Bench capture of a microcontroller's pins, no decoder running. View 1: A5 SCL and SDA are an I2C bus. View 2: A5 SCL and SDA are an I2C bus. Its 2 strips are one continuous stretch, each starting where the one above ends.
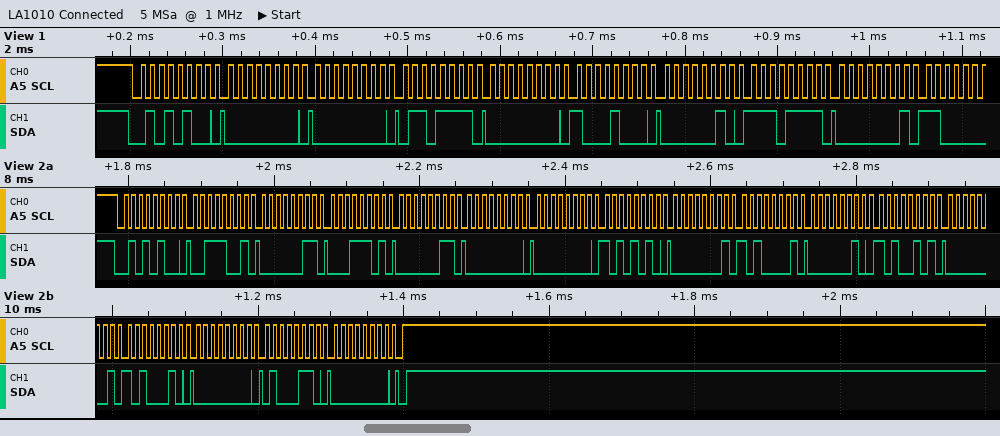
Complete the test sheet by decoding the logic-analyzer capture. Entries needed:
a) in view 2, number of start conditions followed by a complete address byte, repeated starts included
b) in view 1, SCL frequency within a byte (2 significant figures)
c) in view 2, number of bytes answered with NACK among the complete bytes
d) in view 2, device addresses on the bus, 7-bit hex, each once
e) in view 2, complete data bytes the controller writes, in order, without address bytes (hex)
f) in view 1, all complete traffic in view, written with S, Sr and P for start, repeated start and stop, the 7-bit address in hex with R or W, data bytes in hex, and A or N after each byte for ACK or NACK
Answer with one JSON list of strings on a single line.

["1", "100 kHz", "0", "0x2A", "39 03 1D 03 00 00 AA 01 A1 02 A5 01 A2 00 46 00", "S 2AW A 00 A 00 A 6F A 00 A 88 A 02 A EF A 01 A"]
